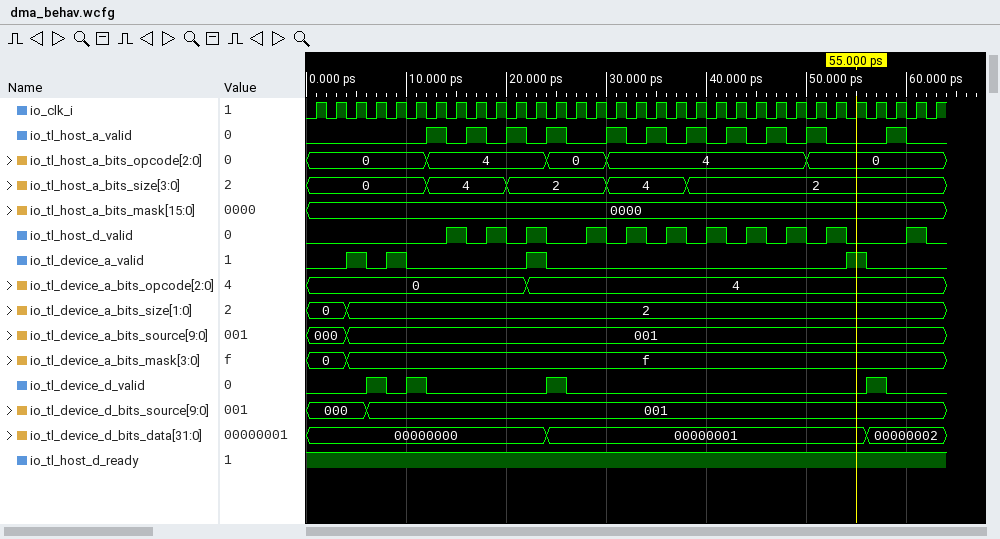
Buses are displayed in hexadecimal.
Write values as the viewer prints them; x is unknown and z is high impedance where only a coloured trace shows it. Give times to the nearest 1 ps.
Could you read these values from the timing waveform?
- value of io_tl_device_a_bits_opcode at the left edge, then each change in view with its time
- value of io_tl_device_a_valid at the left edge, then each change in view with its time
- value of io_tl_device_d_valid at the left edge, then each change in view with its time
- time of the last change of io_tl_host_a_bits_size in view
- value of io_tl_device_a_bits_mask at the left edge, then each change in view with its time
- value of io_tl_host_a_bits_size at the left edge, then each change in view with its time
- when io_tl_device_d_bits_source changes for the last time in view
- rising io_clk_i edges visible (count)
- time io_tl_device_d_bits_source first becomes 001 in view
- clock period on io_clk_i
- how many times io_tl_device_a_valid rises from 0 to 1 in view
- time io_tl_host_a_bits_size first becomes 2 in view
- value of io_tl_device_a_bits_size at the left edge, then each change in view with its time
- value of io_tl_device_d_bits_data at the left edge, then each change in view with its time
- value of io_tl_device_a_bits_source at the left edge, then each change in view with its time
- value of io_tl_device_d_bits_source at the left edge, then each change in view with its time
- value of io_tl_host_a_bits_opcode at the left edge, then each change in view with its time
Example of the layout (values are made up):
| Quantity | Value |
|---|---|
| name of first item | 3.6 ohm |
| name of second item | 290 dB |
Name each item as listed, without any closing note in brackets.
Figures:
| Quantity | Value |
|---|---|
| value of io_tl_device_a_bits_opcode at the left edge, then each change in view with its time | 0, 4 at 22 ps |
| value of io_tl_device_a_valid at the left edge, then each change in view with its time | 0, 1 at 4 ps, 0 at 6 ps, 1 at 8 ps, 0 at 10 ps, 1 at 22 ps, 0 at 24 ps, 1 at 54 ps, 0 at 56 ps |
| value of io_tl_device_d_valid at the left edge, then each change in view with its time | 0, 1 at 6 ps, 0 at 8 ps, 1 at 10 ps, 0 at 12 ps, 1 at 24 ps, 0 at 26 ps, 1 at 56 ps, 0 at 58 ps |
| time of the last change of io_tl_host_a_bits_size in view | 38 ps |
| value of io_tl_device_a_bits_mask at the left edge, then each change in view with its time | 0, f at 4 ps |
| value of io_tl_host_a_bits_size at the left edge, then each change in view with its time | 0, 4 at 12 ps, 2 at 20 ps, 4 at 30 ps, 2 at 38 ps |
| when io_tl_device_d_bits_source changes for the last time in view | 6 ps |
| rising io_clk_i edges visible | 32 |
| time io_tl_device_d_bits_source first becomes 001 in view | 6 ps |
| clock period on io_clk_i | 2 ps |
| how many times io_tl_device_a_valid rises from 0 to 1 in view | 4 |
| time io_tl_host_a_bits_size first becomes 2 in view | 20 ps |
| value of io_tl_device_a_bits_size at the left edge, then each change in view with its time | 0, 2 at 4 ps |
| value of io_tl_device_d_bits_data at the left edge, then each change in view with its time | 00000000, 00000001 at 24 ps, 00000002 at 56 ps |
| value of io_tl_device_a_bits_source at the left edge, then each change in view with its time | 000, 001 at 4 ps |
| value of io_tl_device_d_bits_source at the left edge, then each change in view with its time | 000, 001 at 6 ps |
| value of io_tl_host_a_bits_opcode at the left edge, then each change in view with its time | 0, 4 at 12 ps, 0 at 24 ps, 4 at 30 ps, 0 at 50 ps |
